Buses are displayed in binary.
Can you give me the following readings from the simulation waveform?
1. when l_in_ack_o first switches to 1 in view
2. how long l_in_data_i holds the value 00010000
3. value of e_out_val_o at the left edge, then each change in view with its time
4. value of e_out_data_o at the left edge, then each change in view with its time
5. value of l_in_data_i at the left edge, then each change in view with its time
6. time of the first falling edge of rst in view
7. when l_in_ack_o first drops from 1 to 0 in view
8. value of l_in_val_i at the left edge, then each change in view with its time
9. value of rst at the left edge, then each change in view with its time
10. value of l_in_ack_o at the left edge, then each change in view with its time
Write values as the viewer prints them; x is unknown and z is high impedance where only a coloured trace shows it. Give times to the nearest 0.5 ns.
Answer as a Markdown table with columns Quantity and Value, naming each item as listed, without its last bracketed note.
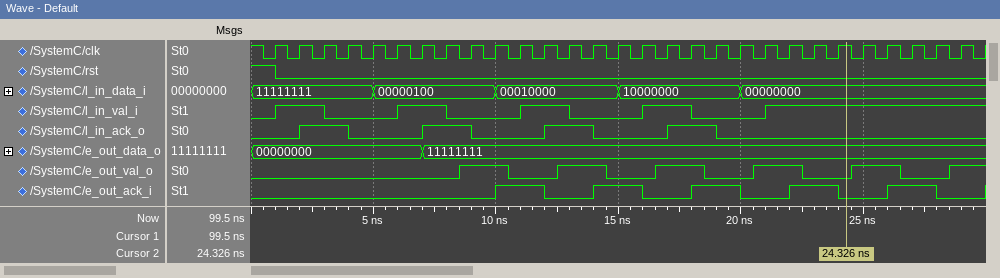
| Quantity | Value |
|---|---|
| when l_in_ack_o first switches to 1 in view | 2 ns |
| how long l_in_data_i holds the value 00010000 | 5 ns |
| value of e_out_val_o at the left edge, then each change in view with its time | 0, 1 at 8.5 ns, 0 at 10.5 ns, 1 at 12.5 ns, 0 at 14.5 ns, 1 at 16.5 ns, 0 at 18.5 ns, 1 at 20.5 ns, 0 at 22.5 ns, 1 at 24.5 ns, 0 at 26.5 ns, 1 at 28.5 ns |
| value of e_out_data_o at the left edge, then each change in view with its time | 00000000, 11111111 at 7 ns |
| value of l_in_data_i at the left edge, then each change in view with its time | 11111111, 00000100 at 5 ns, 00010000 at 10 ns, 10000000 at 15 ns, 00000000 at 20 ns |
| time of the first falling edge of rst in view | 1 ns |
| when l_in_ack_o first drops from 1 to 0 in view | 4 ns |
| value of l_in_val_i at the left edge, then each change in view with its time | 0, 1 at 1 ns, 0 at 3 ns, 1 at 6 ns, 0 at 8 ns, 1 at 11 ns, 0 at 13 ns, 1 at 16 ns, 0 at 18 ns, 1 at 21 ns |
| value of rst at the left edge, then each change in view with its time | 1, 0 at 1 ns |
| value of l_in_ack_o at the left edge, then each change in view with its time | 0, 1 at 2 ns, 0 at 4 ns, 1 at 7 ns, 0 at 9 ns, 1 at 12 ns, 0 at 14 ns, 1 at 17 ns, 0 at 19 ns |
